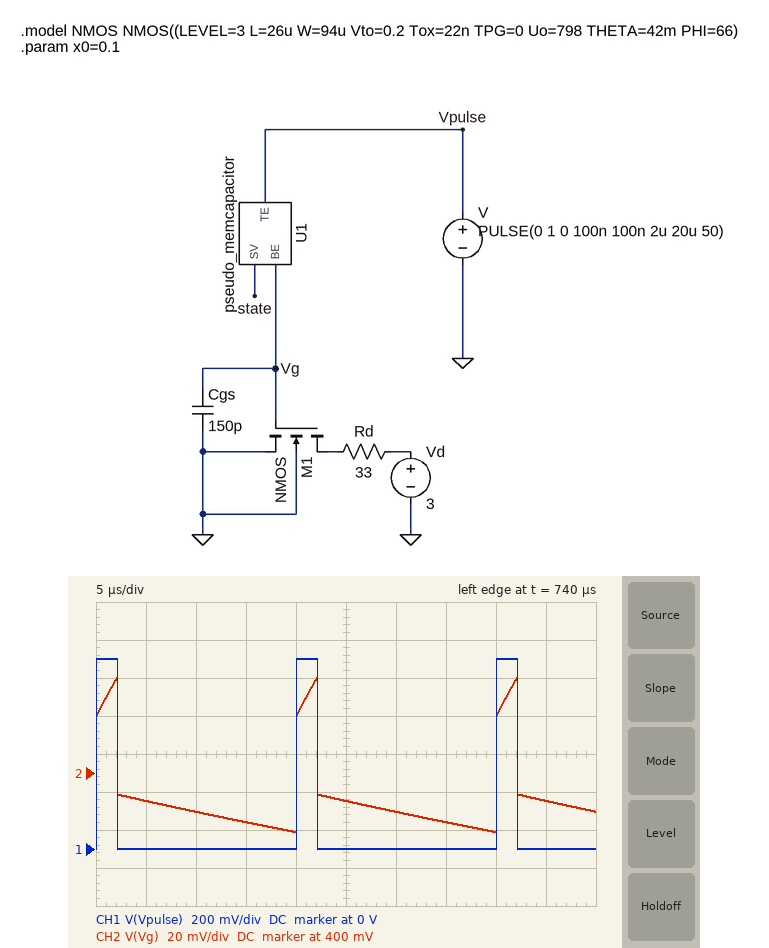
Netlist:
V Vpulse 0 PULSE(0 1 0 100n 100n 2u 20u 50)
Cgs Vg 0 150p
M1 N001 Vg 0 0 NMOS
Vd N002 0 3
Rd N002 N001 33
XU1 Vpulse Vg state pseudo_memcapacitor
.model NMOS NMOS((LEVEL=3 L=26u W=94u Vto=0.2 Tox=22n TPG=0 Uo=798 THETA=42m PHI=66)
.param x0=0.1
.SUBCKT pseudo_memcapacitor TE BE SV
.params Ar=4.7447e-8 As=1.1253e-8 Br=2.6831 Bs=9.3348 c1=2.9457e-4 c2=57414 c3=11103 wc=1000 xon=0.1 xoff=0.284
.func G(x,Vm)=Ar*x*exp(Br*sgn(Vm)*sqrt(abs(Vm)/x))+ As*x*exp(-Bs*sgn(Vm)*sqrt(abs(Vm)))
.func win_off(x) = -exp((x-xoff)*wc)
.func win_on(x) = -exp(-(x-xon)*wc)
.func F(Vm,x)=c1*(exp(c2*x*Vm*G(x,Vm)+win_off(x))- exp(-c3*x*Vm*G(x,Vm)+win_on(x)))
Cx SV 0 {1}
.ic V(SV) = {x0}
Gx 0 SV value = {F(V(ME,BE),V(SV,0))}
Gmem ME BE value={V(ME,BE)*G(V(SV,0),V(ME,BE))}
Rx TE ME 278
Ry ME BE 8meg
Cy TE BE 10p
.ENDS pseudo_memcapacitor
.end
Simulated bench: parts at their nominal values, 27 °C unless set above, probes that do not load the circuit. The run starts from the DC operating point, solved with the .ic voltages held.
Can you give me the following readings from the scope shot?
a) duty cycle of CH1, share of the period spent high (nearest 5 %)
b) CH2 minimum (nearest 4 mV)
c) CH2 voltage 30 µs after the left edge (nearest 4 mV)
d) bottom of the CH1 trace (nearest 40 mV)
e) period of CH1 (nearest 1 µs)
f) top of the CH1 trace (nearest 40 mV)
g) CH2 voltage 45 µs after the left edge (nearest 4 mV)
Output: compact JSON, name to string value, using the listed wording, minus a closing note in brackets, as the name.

{"duty cycle of CH1, share of the period spent high": "10 %", "CH2 minimum": "368 mV", "CH2 voltage 30 µs after the left edge": "380 mV", "bottom of the CH1 trace": "0 V", "period of CH1": "20 µs", "top of the CH1 trace": "1.00 V", "CH2 voltage 45 µs after the left edge": "384 mV"}
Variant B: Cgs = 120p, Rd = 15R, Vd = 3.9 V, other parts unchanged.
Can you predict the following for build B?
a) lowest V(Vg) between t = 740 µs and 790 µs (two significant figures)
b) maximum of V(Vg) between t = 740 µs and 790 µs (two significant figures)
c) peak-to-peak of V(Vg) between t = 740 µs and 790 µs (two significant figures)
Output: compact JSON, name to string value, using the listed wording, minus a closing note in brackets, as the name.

{"lowest V(Vg) between t = 740 µs and 790 µs": "360 mV", "maximum of V(Vg) between t = 740 µs and 790 µs": "460 mV", "peak-to-peak of V(Vg) between t = 740 µs and 790 µs": "98 mV"}
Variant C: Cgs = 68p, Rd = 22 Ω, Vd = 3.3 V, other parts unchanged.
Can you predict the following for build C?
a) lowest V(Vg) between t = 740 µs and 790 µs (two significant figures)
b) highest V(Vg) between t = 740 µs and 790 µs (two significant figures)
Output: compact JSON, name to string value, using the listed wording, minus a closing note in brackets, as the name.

{"lowest V(Vg) between t = 740 µs and 790 µs": "330 mV", "highest V(Vg) between t = 740 µs and 790 µs": "490 mV"}
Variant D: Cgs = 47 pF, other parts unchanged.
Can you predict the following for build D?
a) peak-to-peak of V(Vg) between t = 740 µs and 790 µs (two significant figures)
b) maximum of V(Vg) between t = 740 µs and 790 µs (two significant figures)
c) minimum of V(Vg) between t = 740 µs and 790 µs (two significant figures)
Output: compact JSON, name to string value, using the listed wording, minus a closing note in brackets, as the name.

{"peak-to-peak of V(Vg) between t = 740 µs and 790 µs": "200 mV", "maximum of V(Vg) between t = 740 µs and 790 µs": "510 mV", "minimum of V(Vg) between t = 740 µs and 790 µs": "310 mV"}
